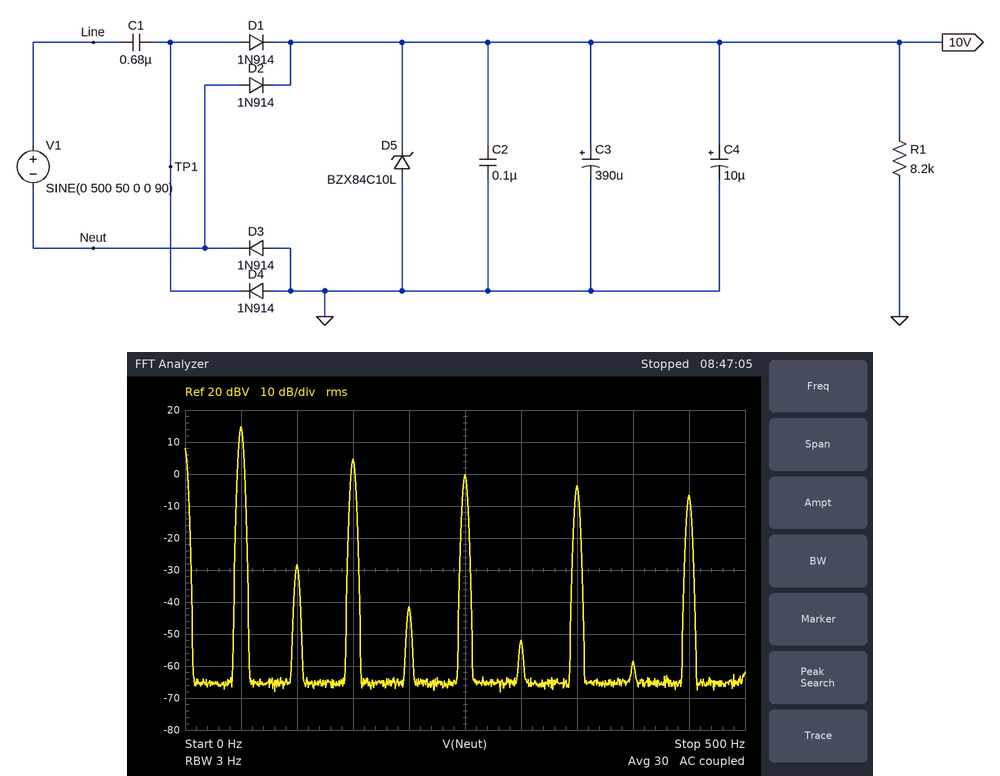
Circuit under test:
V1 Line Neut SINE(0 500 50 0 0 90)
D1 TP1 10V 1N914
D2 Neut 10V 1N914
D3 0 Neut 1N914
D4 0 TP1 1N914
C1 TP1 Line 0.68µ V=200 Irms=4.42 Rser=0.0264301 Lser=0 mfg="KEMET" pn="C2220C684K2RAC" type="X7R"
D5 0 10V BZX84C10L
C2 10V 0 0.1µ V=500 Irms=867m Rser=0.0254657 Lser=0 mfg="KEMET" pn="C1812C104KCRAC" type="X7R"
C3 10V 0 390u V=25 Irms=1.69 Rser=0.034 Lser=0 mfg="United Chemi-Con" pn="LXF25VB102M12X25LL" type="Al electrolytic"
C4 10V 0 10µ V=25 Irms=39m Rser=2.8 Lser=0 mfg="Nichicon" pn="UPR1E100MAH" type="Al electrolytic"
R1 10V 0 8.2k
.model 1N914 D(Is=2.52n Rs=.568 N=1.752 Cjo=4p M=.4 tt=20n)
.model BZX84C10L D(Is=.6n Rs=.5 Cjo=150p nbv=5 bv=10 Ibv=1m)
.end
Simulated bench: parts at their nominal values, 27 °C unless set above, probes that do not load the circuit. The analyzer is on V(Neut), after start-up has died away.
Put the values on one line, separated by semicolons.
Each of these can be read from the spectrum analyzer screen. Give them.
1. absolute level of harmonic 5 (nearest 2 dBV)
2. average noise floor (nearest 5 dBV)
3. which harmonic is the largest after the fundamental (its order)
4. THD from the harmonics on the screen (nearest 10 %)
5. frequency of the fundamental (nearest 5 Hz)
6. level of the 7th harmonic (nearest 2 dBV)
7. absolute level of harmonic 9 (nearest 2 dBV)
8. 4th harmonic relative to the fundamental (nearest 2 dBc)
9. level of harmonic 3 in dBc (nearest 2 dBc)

0 dBV; -65 dBV; 3; 40 %; 50 Hz; -4 dBV; -6 dBV; -56 dBc; -10 dBc
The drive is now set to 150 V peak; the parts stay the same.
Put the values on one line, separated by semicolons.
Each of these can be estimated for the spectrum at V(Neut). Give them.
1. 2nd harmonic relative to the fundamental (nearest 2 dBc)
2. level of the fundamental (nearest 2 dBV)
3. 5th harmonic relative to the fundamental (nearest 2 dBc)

-48 dBc; 14 dBV; -16 dBc
